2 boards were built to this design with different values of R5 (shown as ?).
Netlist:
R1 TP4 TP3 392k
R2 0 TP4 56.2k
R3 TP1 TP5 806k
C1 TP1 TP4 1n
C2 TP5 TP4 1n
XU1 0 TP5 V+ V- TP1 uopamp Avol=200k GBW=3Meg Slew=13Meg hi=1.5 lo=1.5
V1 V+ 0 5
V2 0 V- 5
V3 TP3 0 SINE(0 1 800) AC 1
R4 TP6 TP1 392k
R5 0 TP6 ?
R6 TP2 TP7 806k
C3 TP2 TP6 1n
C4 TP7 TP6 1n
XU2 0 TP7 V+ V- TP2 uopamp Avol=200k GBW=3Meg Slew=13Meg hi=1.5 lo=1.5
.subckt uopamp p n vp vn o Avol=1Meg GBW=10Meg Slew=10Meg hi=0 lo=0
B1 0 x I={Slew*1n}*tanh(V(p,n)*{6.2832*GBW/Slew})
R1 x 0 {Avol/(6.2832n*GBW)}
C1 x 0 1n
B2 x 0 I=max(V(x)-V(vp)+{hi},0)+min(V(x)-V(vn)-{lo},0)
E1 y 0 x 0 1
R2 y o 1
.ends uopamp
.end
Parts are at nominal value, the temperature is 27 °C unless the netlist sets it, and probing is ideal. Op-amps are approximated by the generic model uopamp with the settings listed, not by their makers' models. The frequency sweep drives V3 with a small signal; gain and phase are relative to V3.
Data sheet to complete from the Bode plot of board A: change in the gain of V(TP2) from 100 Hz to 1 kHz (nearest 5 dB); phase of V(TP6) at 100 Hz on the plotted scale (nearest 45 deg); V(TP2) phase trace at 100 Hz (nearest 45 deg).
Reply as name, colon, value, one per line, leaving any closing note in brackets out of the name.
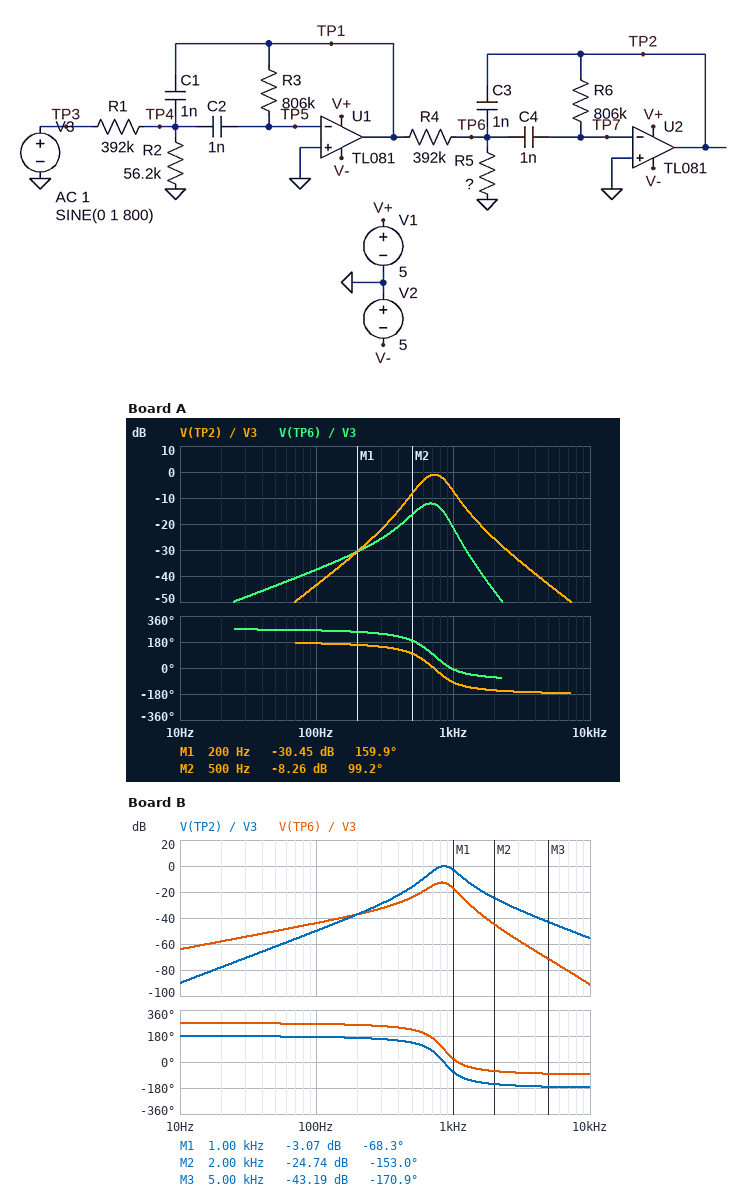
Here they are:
change in the gain of V(TP2) from 100 Hz to 1 kHz: 35 dB
phase of V(TP6) at 100 Hz on the plotted scale: 270 deg
V(TP2) phase trace at 100 Hz: 180 deg
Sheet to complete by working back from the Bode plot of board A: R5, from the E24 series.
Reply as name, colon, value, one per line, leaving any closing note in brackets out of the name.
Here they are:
R5, from the E24 series: 100 kΩ
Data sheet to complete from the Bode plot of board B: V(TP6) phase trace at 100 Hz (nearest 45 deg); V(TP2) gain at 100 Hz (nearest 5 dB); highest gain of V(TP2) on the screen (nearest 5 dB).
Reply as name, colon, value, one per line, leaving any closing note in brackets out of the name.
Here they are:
V(TP6) phase trace at 100 Hz: 270 deg
V(TP2) gain at 100 Hz: -50 dB
highest gain of V(TP2) on the screen: 0 dB
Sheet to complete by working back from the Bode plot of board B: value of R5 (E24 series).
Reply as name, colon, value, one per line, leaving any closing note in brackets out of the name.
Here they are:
value of R5: 43 kΩ
